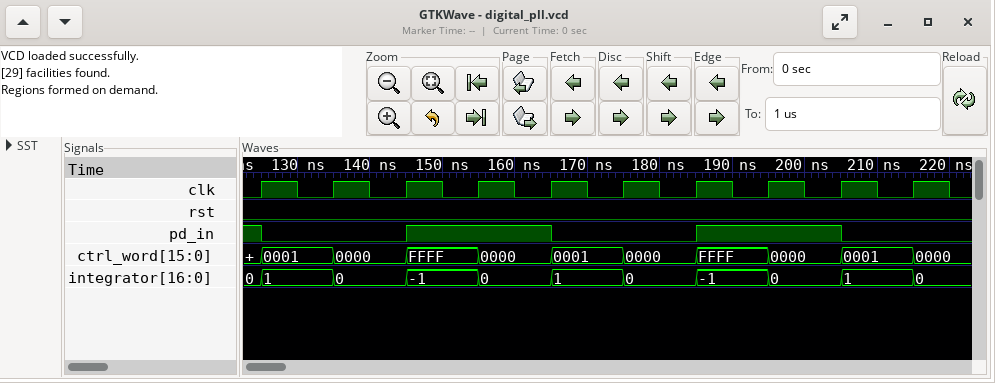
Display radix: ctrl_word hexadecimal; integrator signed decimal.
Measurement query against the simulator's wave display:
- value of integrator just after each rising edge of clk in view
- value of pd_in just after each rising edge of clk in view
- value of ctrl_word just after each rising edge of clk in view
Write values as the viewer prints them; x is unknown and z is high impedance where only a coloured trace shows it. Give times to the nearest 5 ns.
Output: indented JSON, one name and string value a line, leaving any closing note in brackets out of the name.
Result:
{
  "value of integrator just after each rising edge of clk in view": "1, 0, -1, 0, 1, 0, -1, 0, 1, 0",
  "value of pd_in just after each rising edge of clk in view": "0 0 1 1 0 0 1 1 0 0",
  "value of ctrl_word just after each rising edge of clk in view": "0001, 0000, FFFF, 0000, 0001, 0000, FFFF, 0000, 0001, 0000"
}
